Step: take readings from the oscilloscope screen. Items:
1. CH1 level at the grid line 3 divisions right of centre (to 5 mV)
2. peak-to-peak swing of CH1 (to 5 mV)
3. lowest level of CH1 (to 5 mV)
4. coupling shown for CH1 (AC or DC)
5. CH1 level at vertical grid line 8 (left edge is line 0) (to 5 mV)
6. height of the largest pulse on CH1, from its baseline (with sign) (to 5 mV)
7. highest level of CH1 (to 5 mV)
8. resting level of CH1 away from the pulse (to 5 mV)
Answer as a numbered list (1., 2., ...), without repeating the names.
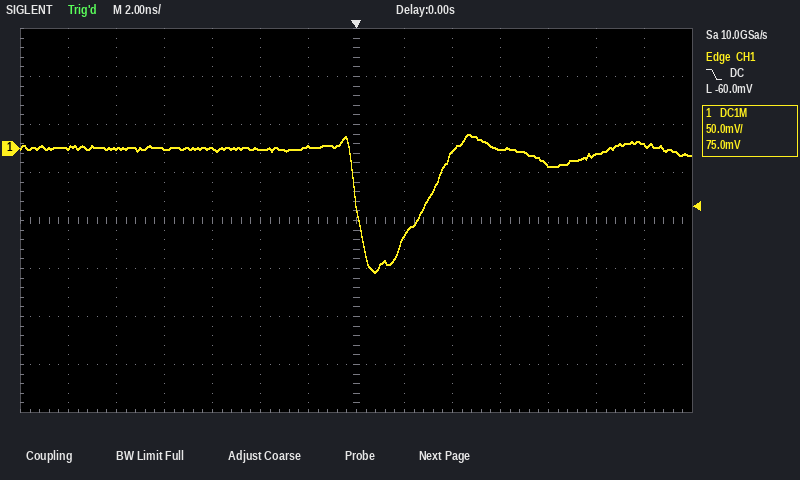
1. 0 mV
2. 145 mV
3. -130 mV
4. DC
5. -90 mV
6. -130 mV
7. 15 mV
8. 0 mV
